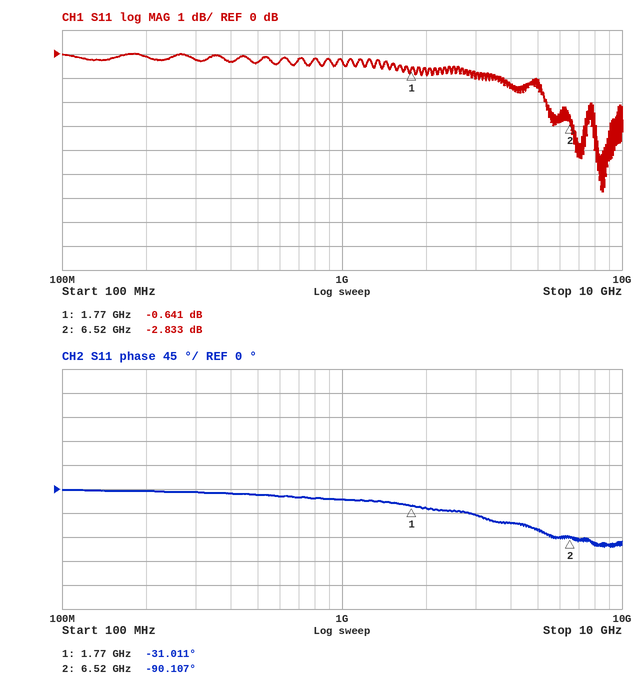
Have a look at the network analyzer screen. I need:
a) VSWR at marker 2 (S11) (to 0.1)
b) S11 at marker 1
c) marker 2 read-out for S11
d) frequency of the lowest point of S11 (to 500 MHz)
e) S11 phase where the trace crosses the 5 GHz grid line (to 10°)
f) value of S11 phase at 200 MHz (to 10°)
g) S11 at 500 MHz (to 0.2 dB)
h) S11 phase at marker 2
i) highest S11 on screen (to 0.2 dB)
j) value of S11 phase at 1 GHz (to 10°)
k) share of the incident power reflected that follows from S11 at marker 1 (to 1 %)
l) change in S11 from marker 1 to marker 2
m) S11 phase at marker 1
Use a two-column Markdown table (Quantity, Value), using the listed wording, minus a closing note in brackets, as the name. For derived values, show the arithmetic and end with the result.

| Quantity | Value |
|---|---|
| VSWR at marker 2 (S11) | (1 + 0.7217)/(1 − 0.7217) ≈ 6.2 |
| S11 at marker 1 | -0.641 dB |
| marker 2 read-out for S11 | -2.833 dB |
| frequency of the lowest point of S11 | 8.5 GHz |
| S11 phase where the trace crosses the 5 GHz grid line | -80° |
| value of S11 phase at 200 MHz | 0° |
| S11 at 500 MHz | -0.4 dB |
| S11 phase at marker 2 | -90.107° |
| highest S11 on screen | 0.0 dB |
| value of S11 phase at 1 GHz | -20° |
| share of the incident power reflected that follows from S11 at marker 1 | 10^(-0.641/10) ≈ 86 % |
| change in S11 from marker 1 to marker 2 | -2.833 − (-0.641) = -2.192 dB |
| S11 phase at marker 1 | -31.011° |
